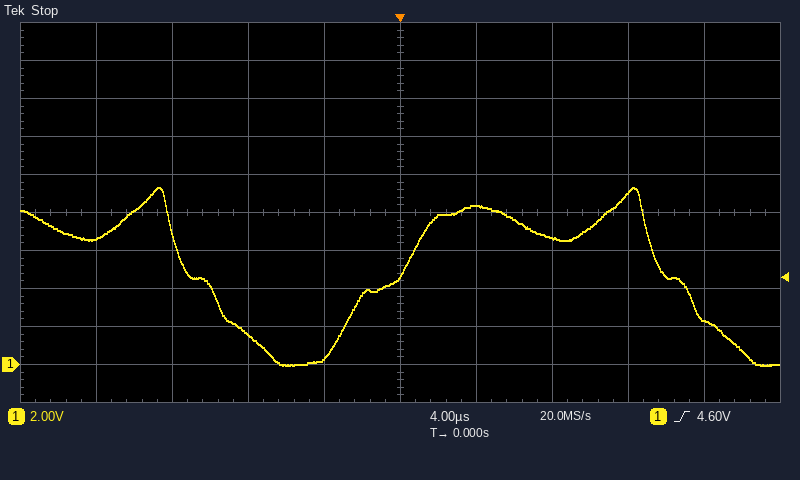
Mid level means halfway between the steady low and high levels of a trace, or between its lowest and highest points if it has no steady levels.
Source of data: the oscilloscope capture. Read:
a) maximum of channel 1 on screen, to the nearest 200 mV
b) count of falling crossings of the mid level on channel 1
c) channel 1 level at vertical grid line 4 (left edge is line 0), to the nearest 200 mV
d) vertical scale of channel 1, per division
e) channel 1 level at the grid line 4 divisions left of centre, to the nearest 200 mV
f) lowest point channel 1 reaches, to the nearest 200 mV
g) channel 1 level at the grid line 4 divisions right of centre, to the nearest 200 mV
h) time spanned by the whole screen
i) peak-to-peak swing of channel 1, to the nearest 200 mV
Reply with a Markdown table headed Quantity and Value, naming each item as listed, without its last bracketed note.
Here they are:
| Quantity | Value |
|---|---|
| maximum of channel 1 on screen, to the nearest 200 mV | 9.4 V |
| count of falling crossings of the mid level on channel 1 | 2 |
| channel 1 level at vertical grid line 4 (left edge is line 0), to the nearest 200 mV | 400 mV |
| vertical scale of channel 1, per division | 2 V |
| channel 1 level at the grid line 4 divisions left of centre, to the nearest 200 mV | 6.6 V |
| lowest point channel 1 reaches, to the nearest 200 mV | 0.0 V |
| channel 1 level at the grid line 4 divisions right of centre, to the nearest 200 mV | 2.4 V |
| time spanned by the whole screen | 40 µs |
| peak-to-peak swing of channel 1, to the nearest 200 mV | 9.4 V |
